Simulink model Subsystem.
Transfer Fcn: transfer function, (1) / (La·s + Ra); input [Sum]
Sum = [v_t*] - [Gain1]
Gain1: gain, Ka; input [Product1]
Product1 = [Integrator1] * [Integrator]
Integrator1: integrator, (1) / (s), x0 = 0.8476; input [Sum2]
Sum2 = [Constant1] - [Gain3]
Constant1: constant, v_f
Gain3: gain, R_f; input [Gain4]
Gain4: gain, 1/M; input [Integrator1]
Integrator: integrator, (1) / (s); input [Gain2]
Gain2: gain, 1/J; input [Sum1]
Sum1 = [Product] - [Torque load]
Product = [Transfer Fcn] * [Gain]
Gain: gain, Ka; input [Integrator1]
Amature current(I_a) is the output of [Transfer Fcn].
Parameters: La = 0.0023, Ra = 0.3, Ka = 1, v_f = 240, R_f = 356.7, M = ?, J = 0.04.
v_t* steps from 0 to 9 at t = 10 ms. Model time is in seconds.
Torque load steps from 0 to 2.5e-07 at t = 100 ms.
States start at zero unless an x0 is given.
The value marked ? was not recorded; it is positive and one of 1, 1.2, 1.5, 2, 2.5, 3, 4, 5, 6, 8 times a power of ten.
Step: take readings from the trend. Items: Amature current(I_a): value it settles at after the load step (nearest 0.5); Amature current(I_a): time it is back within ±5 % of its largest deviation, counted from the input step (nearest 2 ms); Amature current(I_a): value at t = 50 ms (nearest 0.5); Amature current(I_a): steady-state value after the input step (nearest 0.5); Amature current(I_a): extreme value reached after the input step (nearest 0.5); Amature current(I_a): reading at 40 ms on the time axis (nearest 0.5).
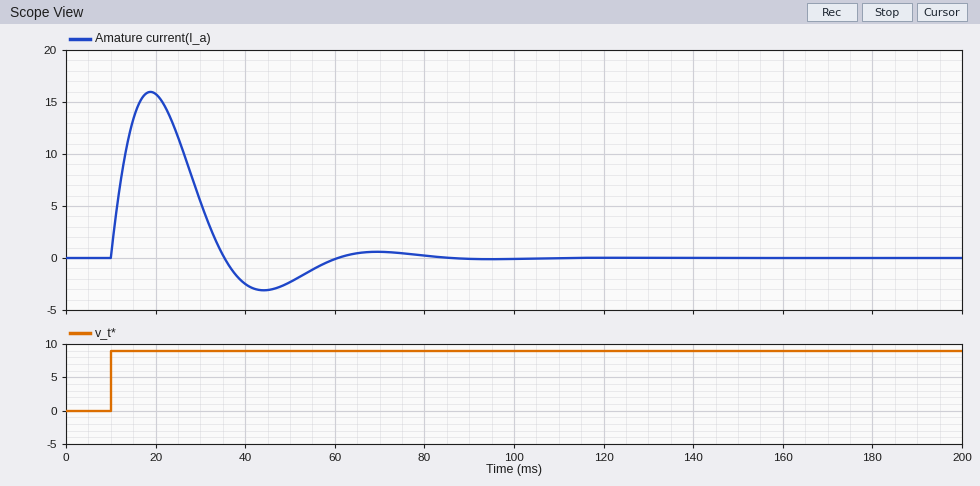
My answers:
0.0
46 ms
-2.5
0.0
16.0
-2.5
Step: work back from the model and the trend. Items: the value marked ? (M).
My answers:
2
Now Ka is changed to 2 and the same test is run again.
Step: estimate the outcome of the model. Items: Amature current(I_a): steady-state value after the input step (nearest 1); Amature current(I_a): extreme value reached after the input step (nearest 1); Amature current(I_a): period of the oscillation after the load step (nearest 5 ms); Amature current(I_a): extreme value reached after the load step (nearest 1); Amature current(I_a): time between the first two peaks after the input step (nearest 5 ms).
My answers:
0
10
25 ms
0
25 ms
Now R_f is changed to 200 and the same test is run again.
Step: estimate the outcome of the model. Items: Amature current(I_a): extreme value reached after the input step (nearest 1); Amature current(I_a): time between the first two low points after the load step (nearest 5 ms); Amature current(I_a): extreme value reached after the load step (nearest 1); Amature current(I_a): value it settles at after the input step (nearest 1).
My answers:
12
25 ms
0
0
